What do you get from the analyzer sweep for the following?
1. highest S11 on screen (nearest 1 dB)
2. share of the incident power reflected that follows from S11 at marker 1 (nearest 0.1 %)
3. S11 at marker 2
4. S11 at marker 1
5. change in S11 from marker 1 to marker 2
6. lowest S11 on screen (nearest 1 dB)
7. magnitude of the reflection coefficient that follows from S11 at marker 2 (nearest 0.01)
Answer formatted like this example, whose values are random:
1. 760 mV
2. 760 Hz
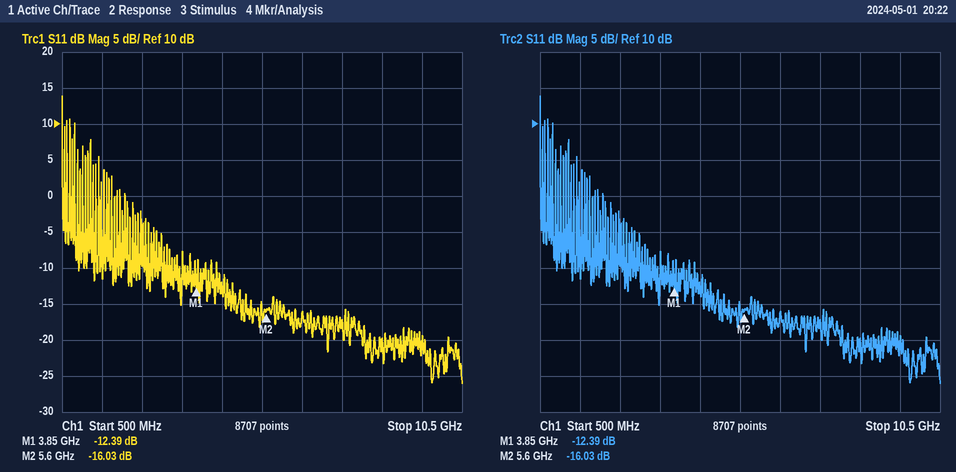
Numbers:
1. 14 dB
2. 5.8 %
3. -16.03 dB
4. -12.39 dB
5. -3.64 dB
6. -26 dB
7. 0.16
